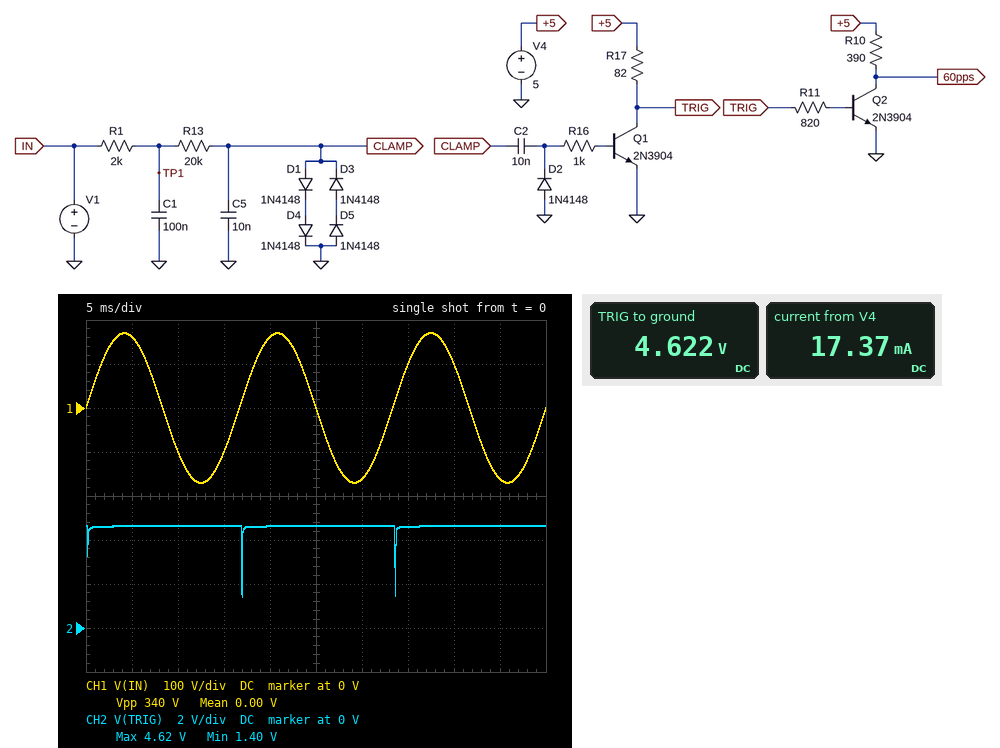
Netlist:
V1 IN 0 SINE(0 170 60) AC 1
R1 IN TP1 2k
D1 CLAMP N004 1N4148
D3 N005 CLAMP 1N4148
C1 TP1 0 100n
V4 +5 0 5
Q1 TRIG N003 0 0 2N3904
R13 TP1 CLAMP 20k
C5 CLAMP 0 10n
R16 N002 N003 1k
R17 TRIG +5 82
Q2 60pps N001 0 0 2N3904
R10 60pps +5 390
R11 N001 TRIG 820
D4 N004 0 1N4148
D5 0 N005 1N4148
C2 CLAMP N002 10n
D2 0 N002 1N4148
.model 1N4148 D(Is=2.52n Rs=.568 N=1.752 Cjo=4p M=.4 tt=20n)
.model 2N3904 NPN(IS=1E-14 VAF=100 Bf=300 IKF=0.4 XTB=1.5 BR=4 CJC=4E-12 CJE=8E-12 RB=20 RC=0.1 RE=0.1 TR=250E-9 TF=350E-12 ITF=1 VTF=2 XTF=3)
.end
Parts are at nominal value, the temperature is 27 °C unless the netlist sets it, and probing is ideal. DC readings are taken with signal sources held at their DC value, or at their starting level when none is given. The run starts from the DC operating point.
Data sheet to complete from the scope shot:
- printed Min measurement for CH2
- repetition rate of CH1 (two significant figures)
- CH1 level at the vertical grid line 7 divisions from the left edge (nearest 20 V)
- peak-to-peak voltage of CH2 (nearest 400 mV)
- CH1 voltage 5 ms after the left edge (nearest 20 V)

1.40 V
60 Hz
100 V
3.2 V
160 V
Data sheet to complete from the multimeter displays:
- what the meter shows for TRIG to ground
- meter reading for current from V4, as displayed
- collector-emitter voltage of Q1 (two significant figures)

4.622 V
17.37 mA
4.6 V
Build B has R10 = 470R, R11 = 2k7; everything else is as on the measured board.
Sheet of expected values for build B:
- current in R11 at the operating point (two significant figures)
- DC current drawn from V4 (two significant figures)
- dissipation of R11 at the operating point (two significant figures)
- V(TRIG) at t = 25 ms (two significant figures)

1.5 mA
12 mA
6.3 mW
4.9 V
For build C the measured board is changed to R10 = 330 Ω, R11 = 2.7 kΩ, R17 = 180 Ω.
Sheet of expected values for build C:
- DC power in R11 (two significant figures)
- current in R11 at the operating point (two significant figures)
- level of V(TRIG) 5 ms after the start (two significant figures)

5.8 mW
1.5 mA
4.7 V
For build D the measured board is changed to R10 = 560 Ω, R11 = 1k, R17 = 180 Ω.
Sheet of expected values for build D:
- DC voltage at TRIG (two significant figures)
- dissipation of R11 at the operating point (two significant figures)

4.4 V
13 mW
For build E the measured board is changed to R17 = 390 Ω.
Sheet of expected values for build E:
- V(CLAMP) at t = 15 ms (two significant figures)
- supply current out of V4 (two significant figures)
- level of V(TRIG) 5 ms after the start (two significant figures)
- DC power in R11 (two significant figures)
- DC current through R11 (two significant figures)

-1.3 V
16 mA
3.6 V
9.8 mW
3.5 mA
